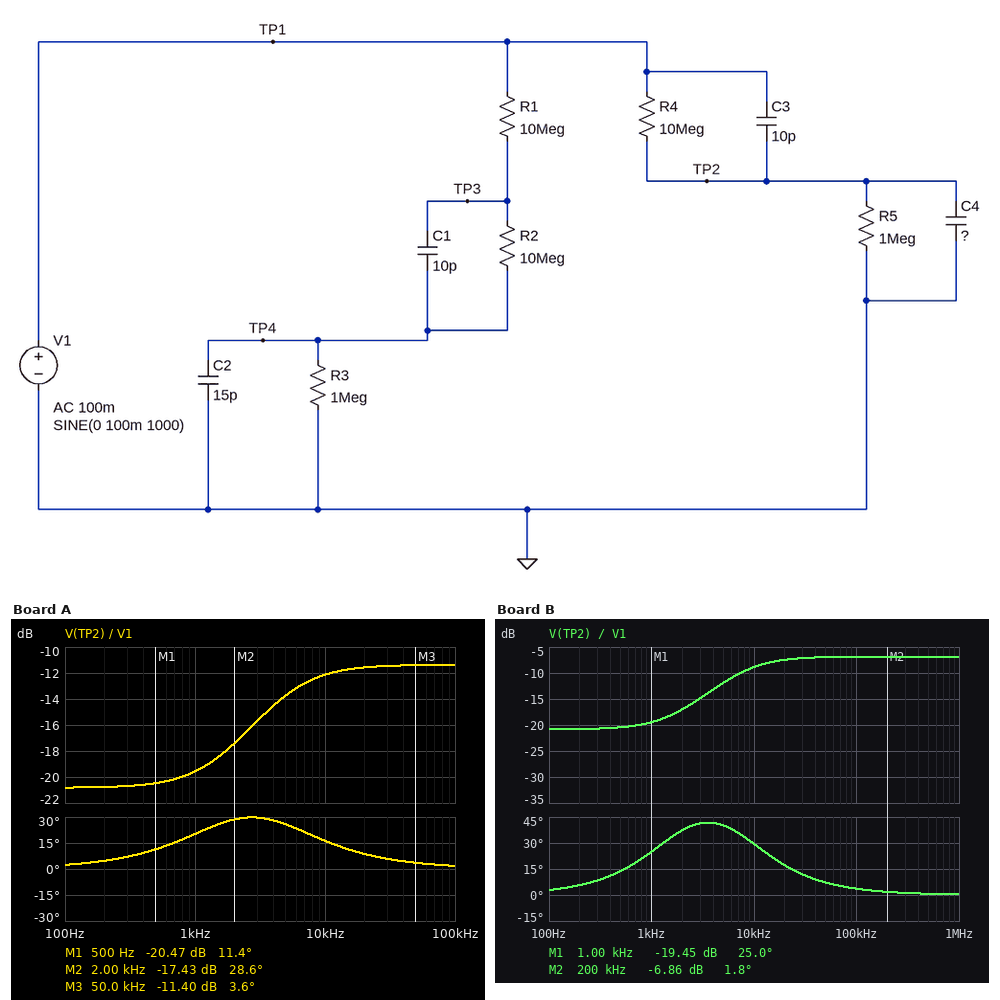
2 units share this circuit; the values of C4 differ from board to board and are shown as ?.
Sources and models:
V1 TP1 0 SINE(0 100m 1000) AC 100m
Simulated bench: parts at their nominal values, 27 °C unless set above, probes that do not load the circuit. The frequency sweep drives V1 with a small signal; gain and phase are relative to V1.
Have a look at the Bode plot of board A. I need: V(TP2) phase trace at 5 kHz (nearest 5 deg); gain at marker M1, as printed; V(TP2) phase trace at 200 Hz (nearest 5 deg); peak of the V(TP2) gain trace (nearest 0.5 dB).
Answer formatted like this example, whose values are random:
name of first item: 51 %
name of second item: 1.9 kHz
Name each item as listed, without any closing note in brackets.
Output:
V(TP2) phase trace at 5 kHz: 25 deg
gain at marker M1, as printed: -20.47 dB
V(TP2) phase trace at 200 Hz: 5 deg
peak of the V(TP2) gain trace: -11.5 dB
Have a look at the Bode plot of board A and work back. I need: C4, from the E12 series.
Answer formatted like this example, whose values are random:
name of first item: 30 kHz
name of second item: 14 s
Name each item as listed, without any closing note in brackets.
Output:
C4, from the E12 series: 27 pF
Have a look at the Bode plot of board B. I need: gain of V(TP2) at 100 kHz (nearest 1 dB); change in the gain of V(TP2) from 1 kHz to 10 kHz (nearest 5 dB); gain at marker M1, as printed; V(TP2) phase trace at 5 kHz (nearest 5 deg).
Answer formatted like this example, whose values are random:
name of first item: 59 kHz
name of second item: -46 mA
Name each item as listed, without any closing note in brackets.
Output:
gain of V(TP2) at 100 kHz: -7 dB
change in the gain of V(TP2) from 1 kHz to 10 kHz: 10 dB
gain at marker M1, as printed: -19.45 dB
V(TP2) phase trace at 5 kHz: 40 deg
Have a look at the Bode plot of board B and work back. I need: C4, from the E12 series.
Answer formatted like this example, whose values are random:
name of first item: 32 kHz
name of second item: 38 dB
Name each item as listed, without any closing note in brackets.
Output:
C4, from the E12 series: 12 pF
